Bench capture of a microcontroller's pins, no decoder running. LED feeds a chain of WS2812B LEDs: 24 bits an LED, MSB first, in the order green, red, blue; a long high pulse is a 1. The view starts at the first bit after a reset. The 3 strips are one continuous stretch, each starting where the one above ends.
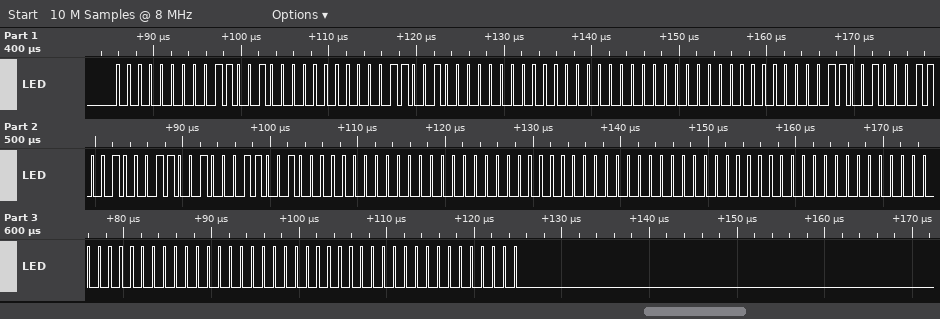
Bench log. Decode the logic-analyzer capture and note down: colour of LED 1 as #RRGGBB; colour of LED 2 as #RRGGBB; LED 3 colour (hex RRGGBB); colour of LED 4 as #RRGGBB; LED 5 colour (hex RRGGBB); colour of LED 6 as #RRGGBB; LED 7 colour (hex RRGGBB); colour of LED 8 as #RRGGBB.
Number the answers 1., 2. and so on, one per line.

1. #640000
2. #006400
3. #000064
4. #646464
5. #000000
6. #000000
7. #000000
8. #000000
